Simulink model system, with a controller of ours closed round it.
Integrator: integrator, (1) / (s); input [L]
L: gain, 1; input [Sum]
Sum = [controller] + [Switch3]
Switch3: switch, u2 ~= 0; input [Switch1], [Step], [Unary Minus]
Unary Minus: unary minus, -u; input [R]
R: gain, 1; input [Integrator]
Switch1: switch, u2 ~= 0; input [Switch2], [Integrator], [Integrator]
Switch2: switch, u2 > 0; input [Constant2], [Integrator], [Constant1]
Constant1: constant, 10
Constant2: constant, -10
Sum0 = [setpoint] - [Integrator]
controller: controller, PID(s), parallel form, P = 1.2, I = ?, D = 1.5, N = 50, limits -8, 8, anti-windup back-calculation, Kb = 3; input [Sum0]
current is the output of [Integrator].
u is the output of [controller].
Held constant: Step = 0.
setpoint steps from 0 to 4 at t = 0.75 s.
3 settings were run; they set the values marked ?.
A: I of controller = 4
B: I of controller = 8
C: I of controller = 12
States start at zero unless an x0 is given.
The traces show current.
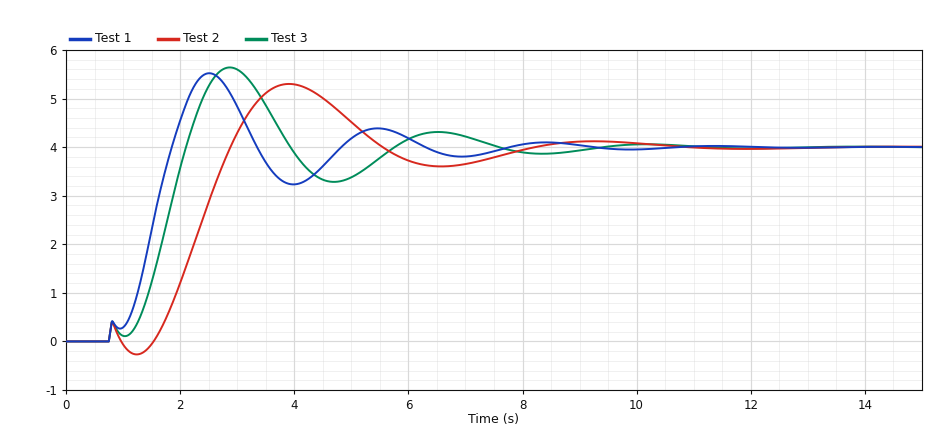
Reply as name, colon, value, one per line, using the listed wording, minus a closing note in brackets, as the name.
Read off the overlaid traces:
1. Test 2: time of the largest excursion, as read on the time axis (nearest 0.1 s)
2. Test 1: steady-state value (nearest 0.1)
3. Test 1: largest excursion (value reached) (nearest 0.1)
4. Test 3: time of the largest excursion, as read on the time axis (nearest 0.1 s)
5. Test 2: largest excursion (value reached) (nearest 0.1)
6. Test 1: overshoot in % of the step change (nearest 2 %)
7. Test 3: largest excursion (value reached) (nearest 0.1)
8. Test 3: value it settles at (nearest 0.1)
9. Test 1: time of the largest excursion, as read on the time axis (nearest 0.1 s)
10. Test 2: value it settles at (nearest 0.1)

Test 2: time of the largest excursion, as read on the time axis: 3.9 s
Test 1: steady-state value: 4.0
Test 1: largest excursion (value reached): 5.5
Test 3: time of the largest excursion, as read on the time axis: 2.9 s
Test 2: largest excursion (value reached): 5.3
Test 1: overshoot in % of the step change: 38 %
Test 3: largest excursion (value reached): 5.6
Test 3: value it settles at: 4.0
Test 1: time of the largest excursion, as read on the time axis: 2.5 s
Test 2: value it settles at: 4.0
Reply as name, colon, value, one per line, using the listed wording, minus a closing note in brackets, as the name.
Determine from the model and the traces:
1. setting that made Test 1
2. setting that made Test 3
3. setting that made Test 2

setting that made Test 1: C
setting that made Test 3: B
setting that made Test 2: A
